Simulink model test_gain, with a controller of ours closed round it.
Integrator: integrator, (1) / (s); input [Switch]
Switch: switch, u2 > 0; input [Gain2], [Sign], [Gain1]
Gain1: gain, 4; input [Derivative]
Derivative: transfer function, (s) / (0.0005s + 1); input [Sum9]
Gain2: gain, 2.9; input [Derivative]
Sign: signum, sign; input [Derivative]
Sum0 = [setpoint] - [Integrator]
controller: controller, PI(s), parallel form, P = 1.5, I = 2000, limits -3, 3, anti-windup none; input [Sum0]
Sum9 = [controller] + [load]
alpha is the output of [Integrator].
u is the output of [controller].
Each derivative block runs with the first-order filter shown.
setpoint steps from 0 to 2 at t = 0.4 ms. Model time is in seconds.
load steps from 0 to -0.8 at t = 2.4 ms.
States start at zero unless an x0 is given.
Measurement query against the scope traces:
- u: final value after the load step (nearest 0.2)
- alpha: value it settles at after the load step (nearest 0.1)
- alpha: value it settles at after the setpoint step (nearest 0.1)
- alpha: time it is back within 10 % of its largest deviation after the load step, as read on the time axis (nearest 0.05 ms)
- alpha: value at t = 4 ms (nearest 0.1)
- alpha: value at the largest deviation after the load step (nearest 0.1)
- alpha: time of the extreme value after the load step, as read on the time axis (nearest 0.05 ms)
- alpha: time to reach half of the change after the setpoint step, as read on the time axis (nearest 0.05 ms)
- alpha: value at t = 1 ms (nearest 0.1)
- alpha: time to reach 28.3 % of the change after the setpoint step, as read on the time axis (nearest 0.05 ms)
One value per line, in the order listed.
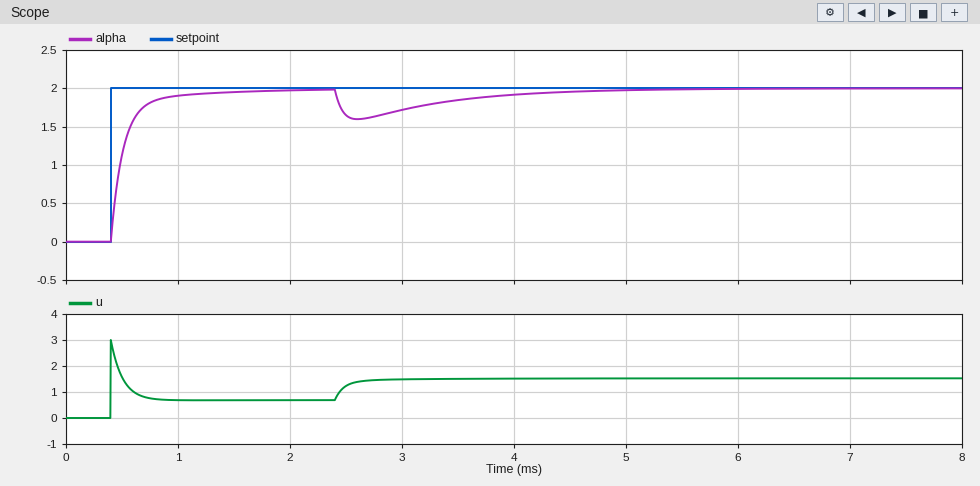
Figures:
1.6
2.0
2.0
4.65 ms
1.9
1.6
2.60 ms
0.50 ms
1.9
0.45 ms
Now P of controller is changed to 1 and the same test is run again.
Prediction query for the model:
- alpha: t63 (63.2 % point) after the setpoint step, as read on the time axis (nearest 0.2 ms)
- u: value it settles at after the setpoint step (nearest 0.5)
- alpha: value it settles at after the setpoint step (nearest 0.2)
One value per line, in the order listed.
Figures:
0.6 ms
0.5
2.0
